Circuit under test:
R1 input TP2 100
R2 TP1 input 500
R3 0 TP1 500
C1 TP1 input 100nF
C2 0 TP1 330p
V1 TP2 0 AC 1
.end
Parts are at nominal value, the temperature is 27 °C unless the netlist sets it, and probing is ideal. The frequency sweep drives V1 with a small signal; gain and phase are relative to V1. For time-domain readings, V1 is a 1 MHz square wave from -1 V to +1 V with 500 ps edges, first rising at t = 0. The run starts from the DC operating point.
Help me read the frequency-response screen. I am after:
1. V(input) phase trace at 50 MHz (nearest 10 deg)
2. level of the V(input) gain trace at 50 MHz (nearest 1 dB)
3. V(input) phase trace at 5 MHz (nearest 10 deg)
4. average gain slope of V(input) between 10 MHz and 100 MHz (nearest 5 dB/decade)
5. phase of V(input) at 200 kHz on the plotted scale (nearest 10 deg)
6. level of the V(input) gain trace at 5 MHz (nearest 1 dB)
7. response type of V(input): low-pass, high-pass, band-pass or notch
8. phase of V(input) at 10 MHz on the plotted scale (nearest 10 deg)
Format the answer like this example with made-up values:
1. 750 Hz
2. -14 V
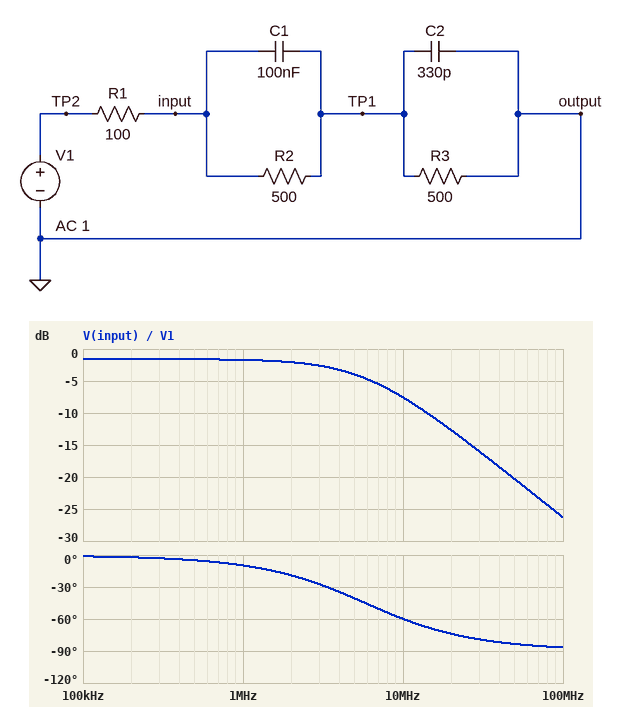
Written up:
1. -80 deg
2. -20 dB
3. -40 deg
4. -20 dB/decade
5. 0 deg
6. -4 dB
7. low-pass
8. -60 deg
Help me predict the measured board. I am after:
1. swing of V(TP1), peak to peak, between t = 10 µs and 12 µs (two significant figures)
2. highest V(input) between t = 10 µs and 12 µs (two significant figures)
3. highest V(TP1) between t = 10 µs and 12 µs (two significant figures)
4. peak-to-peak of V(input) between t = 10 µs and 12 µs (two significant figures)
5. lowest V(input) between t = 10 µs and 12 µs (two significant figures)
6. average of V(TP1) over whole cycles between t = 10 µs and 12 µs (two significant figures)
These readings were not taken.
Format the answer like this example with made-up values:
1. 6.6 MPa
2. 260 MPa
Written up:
1. 1.7 V
2. 790 mV
3. 1.1 V
4. 1.7 V
5. -890 mV
6. 250 mV
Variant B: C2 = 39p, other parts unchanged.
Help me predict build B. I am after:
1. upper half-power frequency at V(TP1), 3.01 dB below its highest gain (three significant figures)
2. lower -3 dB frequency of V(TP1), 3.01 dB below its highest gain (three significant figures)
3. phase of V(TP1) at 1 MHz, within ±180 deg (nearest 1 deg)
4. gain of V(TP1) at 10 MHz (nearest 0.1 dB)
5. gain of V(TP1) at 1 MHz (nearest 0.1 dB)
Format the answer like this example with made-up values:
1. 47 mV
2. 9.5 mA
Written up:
1. 49.0 MHz
2. 3.71 kHz
3. -1 deg
4. -1.8 dB
5. -1.6 dB
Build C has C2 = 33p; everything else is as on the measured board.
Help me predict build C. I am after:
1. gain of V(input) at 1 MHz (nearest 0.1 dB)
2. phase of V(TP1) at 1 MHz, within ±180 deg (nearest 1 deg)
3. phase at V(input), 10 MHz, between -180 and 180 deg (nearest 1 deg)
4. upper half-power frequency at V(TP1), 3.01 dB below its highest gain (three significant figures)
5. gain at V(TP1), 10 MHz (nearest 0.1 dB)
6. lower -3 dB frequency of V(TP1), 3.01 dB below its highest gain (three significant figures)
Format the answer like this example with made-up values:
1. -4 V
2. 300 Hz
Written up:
1. -1.6 dB
2. -1 deg
3. -10 deg
4. 57.9 MHz
5. -1.7 dB
6. 3.71 kHz
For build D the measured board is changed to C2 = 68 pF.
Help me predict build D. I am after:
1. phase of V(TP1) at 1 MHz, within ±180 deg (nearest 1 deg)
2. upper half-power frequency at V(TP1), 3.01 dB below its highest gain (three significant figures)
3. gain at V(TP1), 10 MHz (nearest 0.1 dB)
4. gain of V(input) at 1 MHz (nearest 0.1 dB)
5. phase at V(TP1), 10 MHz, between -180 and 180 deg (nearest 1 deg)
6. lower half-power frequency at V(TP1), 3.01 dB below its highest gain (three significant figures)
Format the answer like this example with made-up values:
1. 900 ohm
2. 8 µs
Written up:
1. -2 deg
2. 28.1 MHz
3. -2.1 dB
4. -1.6 dB
5. -20 deg
6. 3.71 kHz
